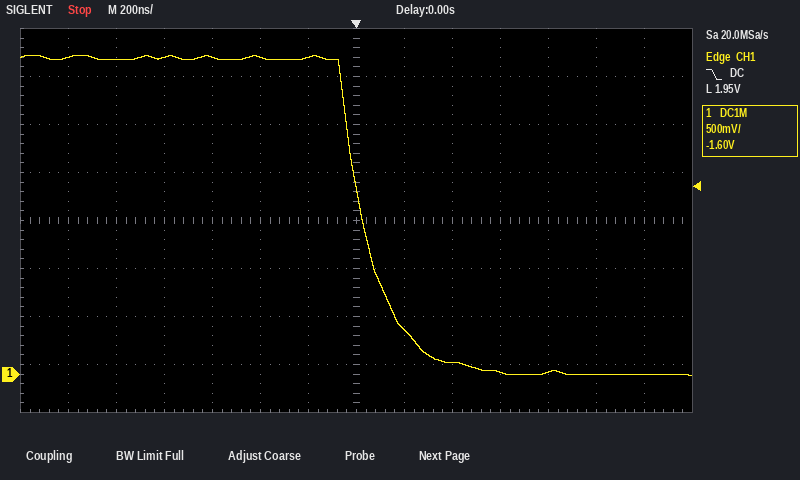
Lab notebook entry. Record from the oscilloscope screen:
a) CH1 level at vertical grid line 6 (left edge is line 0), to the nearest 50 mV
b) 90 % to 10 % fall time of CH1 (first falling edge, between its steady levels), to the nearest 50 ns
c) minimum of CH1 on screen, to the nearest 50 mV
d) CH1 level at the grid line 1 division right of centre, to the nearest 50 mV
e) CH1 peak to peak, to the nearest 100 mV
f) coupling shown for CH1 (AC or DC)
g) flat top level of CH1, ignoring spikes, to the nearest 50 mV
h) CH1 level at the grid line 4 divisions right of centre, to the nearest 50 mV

3.30 V
300 ns
0 mV
450 mV
3.30 V
DC
3.30 V
0 mV
